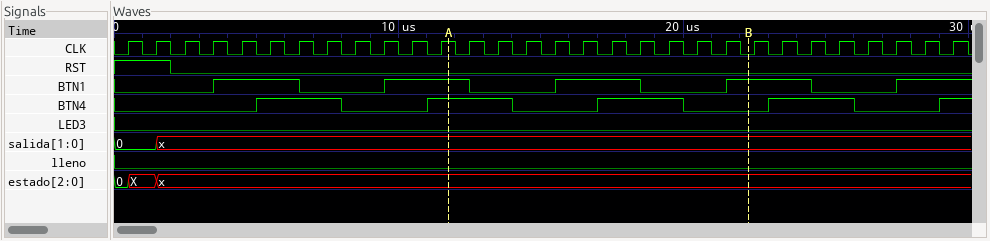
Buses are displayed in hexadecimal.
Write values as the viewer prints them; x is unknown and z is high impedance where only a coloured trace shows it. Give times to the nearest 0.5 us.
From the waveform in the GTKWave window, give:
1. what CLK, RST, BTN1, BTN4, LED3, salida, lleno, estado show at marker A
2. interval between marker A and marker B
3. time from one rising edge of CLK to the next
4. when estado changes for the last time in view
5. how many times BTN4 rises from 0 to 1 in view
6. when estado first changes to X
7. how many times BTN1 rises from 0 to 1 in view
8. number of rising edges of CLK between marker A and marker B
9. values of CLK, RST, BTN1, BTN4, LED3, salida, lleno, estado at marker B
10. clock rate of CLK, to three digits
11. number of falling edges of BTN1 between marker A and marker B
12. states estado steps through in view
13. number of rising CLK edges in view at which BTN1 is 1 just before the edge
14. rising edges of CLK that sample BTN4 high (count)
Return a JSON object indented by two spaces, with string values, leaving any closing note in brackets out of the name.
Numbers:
{
  "what CLK, RST, BTN1, BTN4, LED3, salida, lleno, estado show at marker A": "CLK=1, RST=0, BTN1=1, BTN4=1, LED3=0, salida=x, lleno=0, estado=x",
  "interval between marker A and marker B": "10.5 us",
  "time from one rising edge of CLK to the next": "1 us",
  "when estado changes for the last time in view": "1.5 us",
  "how many times BTN4 rises from 0 to 1 in view": "5",
  "when estado first changes to X": "0.5 us",
  "how many times BTN1 rises from 0 to 1 in view": "5",
  "number of rising edges of CLK between marker A and marker B": "10",
  "values of CLK, RST, BTN1, BTN4, LED3, salida, lleno, estado at marker B": "CLK=0, RST=0, BTN1=1, BTN4=0, LED3=0, salida=x, lleno=0, estado=x",
  "clock rate of CLK, to three digits": "1.00 MHz",
  "number of falling edges of BTN1 between marker A and marker B": "2",
  "states estado steps through in view": "0, X, x",
  "number of rising CLK edges in view at which BTN1 is 1 just before the edge": "14",
  "rising edges of CLK that sample BTN4 high": "13"
}
